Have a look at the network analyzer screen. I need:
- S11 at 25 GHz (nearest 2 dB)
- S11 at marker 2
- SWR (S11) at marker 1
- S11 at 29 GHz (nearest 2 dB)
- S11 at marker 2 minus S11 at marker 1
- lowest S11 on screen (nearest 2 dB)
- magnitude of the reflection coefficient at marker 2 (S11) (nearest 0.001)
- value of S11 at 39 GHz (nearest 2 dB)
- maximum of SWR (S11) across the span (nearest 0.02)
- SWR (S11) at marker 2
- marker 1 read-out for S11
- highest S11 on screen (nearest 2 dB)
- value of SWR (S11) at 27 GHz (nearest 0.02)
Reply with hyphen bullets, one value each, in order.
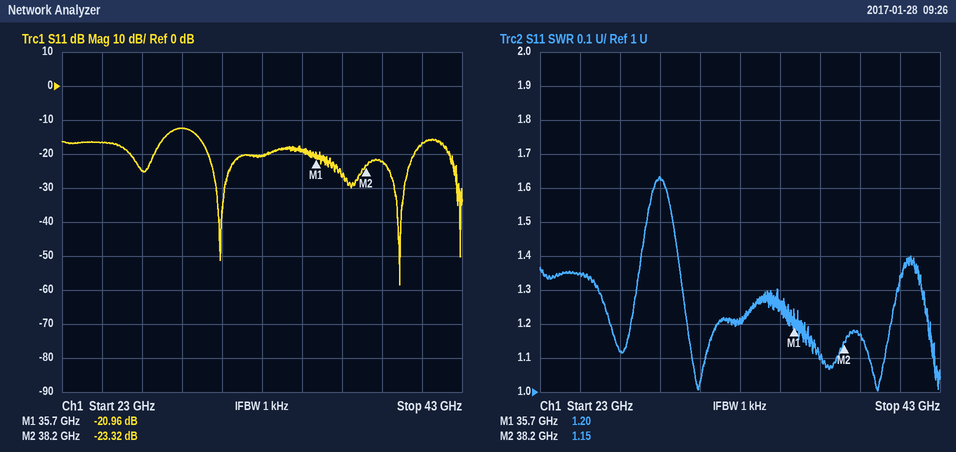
- -16 dB
- -23.32 dB
- 1.20
- -12 dB
- -2.36 dB
- -58 dB
- 0.068
- -22 dB
- 1.64
- 1.15
- -20.96 dB
- -12 dB
- 1.12
